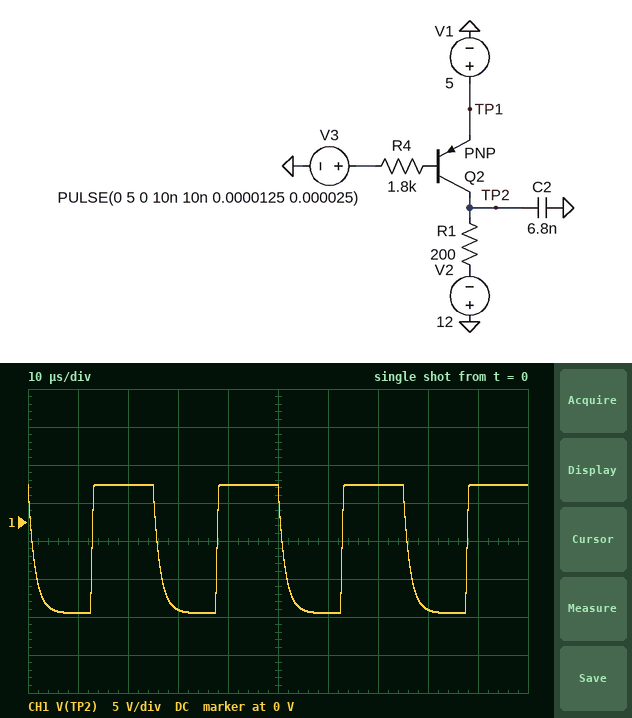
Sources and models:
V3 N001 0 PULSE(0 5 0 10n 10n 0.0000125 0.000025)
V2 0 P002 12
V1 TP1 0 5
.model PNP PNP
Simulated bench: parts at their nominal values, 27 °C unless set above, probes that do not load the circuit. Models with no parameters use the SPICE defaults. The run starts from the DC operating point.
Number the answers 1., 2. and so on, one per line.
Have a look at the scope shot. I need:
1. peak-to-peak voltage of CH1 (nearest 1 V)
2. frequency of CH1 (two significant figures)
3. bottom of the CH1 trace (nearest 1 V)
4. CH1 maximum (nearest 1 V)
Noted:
1. 17 V
2. 40 kHz
3. -12 V
4. 5 V
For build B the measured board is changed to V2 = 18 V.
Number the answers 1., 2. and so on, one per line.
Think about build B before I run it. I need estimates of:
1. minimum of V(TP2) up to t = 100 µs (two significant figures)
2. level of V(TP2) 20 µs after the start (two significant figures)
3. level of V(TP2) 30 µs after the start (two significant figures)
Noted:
1. -18 V
2. 4.9 V
3. -17 V
